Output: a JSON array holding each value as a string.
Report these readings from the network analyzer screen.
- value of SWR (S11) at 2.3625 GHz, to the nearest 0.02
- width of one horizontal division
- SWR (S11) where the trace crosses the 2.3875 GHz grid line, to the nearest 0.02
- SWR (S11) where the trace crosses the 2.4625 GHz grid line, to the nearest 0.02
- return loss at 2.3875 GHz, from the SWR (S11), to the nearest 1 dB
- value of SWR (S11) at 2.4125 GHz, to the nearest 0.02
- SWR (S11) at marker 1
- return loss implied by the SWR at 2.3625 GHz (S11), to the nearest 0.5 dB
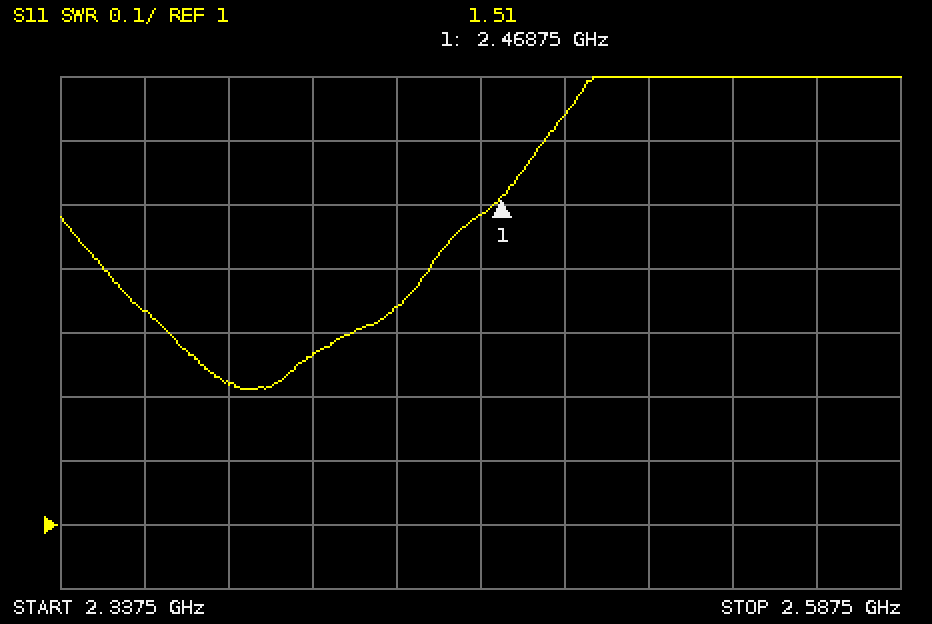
["1.34", "25 MHz", "1.22", "1.48", "20 dB", "1.26", "1.51", "17.0 dB"]
